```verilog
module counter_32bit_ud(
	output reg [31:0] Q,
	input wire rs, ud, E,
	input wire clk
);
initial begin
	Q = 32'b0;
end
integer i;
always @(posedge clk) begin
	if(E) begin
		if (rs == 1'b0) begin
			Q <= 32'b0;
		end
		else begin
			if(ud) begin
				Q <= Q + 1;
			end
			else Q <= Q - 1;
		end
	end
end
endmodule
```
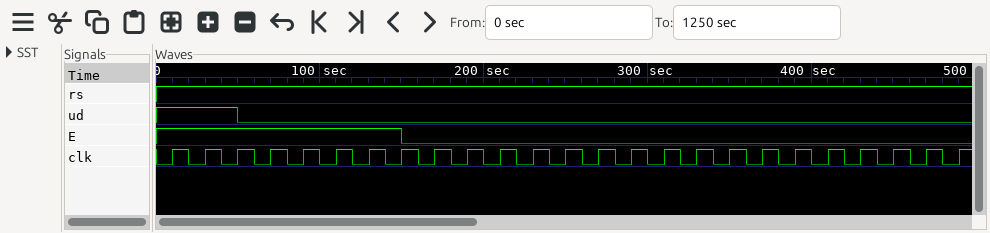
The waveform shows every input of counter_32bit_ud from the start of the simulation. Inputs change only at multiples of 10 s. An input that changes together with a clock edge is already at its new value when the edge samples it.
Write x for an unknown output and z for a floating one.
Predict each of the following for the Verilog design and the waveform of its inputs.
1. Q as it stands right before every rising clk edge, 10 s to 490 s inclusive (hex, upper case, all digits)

00000000, 00000001, 00000002, 00000001, 00000000, FFFFFFFF, FFFFFFFE, FFFFFFFD, FFFFFFFD, FFFFFFFD, FFFFFFFD, FFFFFFFD, FFFFFFFD, FFFFFFFD, FFFFFFFD, FFFFFFFD, FFFFFFFD, FFFFFFFD, FFFFFFFD, FFFFFFFD, FFFFFFFD, FFFFFFFD, FFFFFFFD, FFFFFFFD, FFFFFFFD
